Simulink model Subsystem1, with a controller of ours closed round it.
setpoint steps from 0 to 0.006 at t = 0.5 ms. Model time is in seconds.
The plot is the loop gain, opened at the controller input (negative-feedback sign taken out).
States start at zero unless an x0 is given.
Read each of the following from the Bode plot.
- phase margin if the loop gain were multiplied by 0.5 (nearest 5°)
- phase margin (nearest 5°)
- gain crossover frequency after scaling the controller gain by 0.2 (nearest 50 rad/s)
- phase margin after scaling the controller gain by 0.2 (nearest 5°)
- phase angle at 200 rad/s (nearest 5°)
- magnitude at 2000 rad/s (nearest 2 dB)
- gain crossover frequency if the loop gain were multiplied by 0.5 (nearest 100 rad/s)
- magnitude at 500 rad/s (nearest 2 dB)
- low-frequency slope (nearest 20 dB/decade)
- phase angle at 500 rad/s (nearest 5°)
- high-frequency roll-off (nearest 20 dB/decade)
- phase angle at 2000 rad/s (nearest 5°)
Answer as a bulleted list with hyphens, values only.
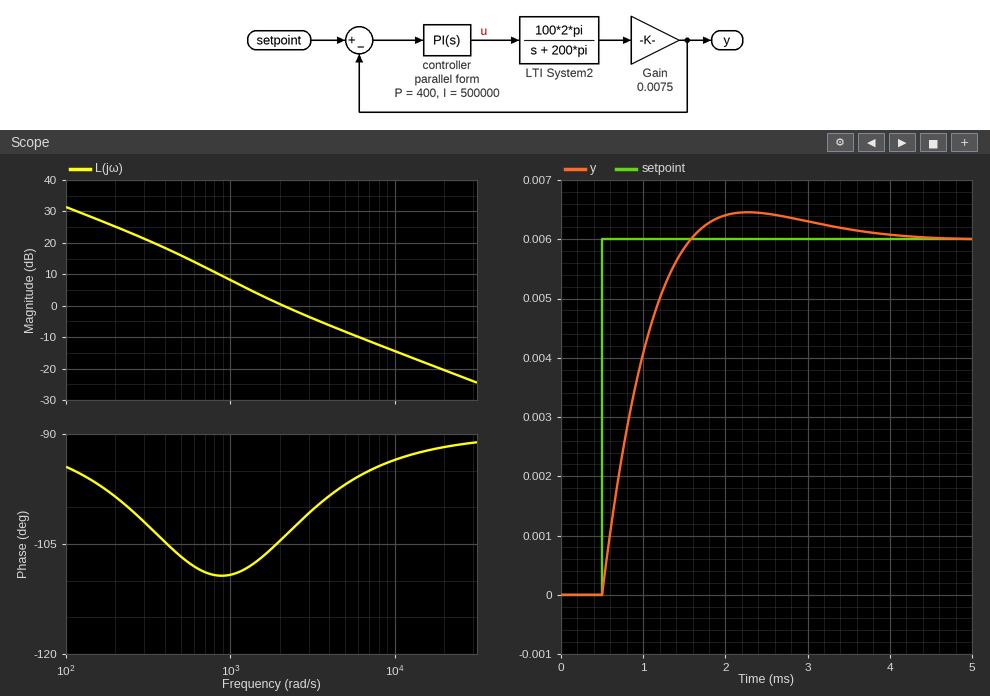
- 70°
- 75°
- 600 rad/s
- 70°
- -100°
- 0 dB
- 1200 rad/s
- 16 dB
- -20 dB/decade
- -105°
- -20 dB/decade
- -105°
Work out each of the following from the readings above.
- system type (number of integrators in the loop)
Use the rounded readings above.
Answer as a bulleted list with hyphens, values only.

- 1
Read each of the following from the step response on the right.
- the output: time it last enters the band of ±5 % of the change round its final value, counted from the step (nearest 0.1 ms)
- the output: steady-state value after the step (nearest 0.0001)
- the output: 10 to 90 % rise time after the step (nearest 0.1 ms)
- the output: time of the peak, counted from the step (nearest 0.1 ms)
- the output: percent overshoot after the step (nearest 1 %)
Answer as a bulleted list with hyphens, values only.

- 2.5 ms
- 0.0060
- 0.8 ms
- 1.8 ms
- 8 %
